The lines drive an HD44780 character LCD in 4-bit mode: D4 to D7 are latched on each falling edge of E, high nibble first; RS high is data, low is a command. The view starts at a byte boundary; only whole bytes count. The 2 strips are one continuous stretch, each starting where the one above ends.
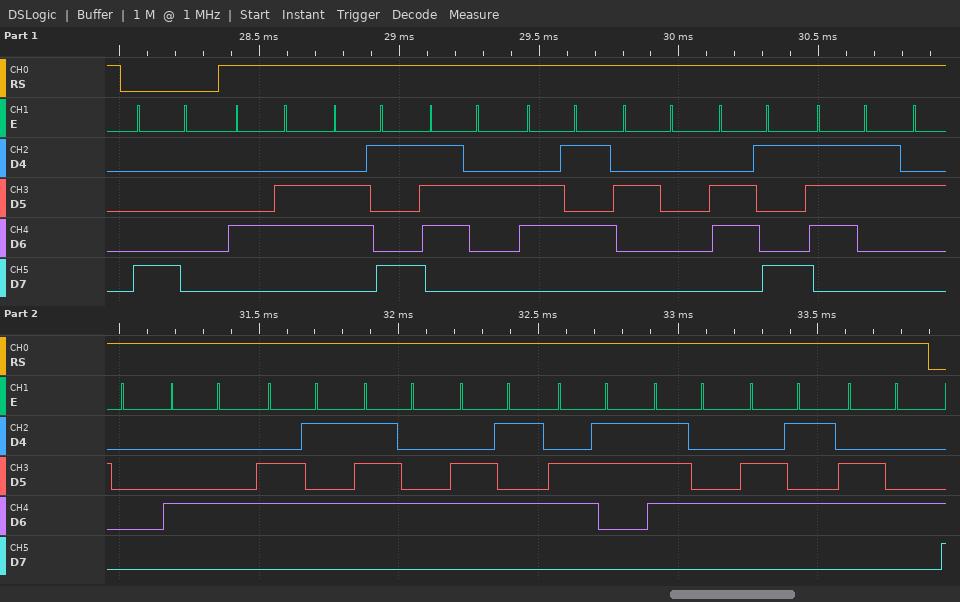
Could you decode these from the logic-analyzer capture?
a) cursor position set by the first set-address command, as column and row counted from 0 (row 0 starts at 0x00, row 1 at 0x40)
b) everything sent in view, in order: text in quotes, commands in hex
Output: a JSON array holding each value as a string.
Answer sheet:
["column 0, row 0", "0x80 \"Fire is Detected\""]
